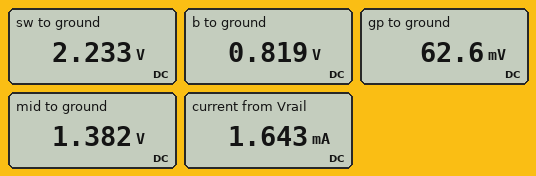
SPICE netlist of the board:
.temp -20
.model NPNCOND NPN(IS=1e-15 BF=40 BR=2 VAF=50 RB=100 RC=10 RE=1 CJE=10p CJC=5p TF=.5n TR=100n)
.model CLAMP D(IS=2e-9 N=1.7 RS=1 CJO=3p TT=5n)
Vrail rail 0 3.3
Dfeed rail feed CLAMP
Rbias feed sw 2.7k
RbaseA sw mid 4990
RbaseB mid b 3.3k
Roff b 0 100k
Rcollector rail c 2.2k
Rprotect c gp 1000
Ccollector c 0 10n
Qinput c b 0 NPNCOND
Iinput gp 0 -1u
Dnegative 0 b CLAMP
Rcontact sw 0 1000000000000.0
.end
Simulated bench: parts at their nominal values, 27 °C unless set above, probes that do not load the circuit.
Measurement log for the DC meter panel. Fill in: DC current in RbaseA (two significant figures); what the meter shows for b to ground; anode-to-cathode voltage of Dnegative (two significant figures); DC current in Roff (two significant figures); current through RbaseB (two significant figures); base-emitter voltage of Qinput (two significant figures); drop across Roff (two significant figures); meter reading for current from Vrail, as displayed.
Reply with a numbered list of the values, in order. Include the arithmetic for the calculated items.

1. (2.233 V - 1.382 V) / 4.99 kΩ = 170 µA
2. 0.819 V
3. 0 V - 819 mV = -820 mV
4. (819 mV) / 100 kΩ = 8.2 µA
5. (1.382 V - 819 mV) / 3.3 kΩ = 170 µA
6. 819 mV = 820 mV
7. 819 mV = 820 mV
8. 1.643 mA
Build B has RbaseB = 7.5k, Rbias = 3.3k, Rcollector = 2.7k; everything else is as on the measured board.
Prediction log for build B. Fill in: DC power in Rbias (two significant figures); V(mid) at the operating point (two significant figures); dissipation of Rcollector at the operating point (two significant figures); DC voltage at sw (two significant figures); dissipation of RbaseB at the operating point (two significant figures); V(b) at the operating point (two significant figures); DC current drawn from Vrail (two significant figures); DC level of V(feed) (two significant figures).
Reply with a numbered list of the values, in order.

1. 48 µW
2. 1.7 V
3. 3.9 mW
4. 2.3 V
5. 110 µW
6. 810 mV
7. 1.3 mA
8. 2.7 V
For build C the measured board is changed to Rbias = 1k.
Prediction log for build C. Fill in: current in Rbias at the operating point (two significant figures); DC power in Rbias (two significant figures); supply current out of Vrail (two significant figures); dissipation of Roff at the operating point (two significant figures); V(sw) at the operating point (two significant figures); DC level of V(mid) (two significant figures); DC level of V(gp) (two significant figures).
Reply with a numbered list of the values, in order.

1. 200 µA
2. 40 µW
3. 1.7 mA
4. 6.8 µW
5. 2.5 V
6. 1.5 V
7. 59 mV
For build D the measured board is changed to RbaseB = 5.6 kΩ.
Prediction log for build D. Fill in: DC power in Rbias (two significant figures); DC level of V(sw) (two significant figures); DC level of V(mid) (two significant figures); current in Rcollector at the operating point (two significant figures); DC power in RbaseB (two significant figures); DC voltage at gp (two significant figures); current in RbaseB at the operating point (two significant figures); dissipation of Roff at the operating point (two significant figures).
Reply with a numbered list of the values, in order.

1. 54 µW
2. 2.3 V
3. 1.6 V
4. 1.5 mA
5. 110 µW
6. 67 mV
7. 140 µA
8. 6.6 µW
